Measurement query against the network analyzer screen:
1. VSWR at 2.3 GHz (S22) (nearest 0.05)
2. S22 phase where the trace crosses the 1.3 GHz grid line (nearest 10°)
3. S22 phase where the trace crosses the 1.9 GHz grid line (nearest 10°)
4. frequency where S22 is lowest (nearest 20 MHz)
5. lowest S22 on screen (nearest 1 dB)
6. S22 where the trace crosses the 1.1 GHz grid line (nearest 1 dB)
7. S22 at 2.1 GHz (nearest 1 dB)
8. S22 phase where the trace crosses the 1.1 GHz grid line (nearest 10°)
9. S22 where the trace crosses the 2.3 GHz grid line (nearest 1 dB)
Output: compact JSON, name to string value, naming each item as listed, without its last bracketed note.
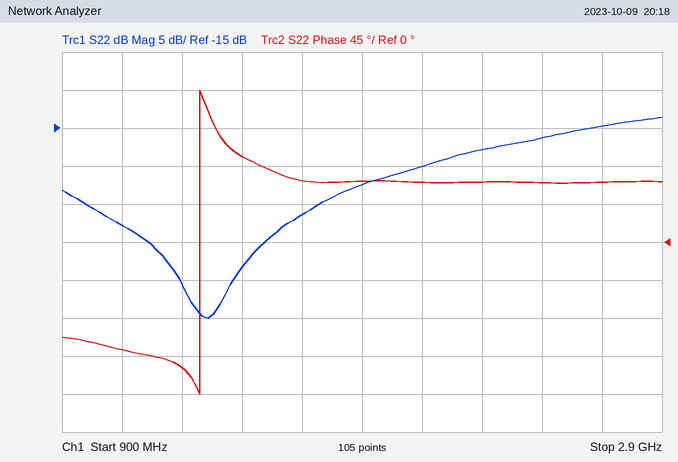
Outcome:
{"VSWR at 2.3 GHz (S22)": "1.30", "S22 phase where the trace crosses the 1.3 GHz grid line": "-150°", "S22 phase where the trace crosses the 1.9 GHz grid line": "70°", "frequency where S22 is lowest": "1.38 GHz", "lowest S22 on screen": "-40 dB", "S22 where the trace crosses the 1.1 GHz grid line": "-28 dB", "S22 at 2.1 GHz": "-20 dB", "S22 phase where the trace crosses the 1.1 GHz grid line": "-130°", "S22 where the trace crosses the 2.3 GHz grid line": "-18 dB"}
